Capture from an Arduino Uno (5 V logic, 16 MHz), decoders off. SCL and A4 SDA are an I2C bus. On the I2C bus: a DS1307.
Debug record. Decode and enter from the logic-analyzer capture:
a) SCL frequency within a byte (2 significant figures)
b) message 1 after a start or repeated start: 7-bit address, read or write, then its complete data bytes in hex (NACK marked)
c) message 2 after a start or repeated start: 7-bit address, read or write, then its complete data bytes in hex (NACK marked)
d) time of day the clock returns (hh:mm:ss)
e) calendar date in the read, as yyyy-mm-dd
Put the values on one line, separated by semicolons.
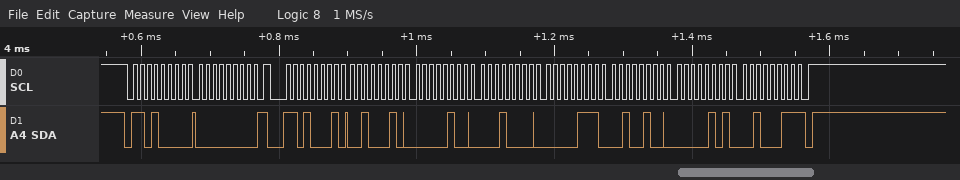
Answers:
100 kHz; 0x68 write: 00; 0x68 read: 22 04 10 07 24 05 23 NACK; 10:04:22; 2023-05-24
